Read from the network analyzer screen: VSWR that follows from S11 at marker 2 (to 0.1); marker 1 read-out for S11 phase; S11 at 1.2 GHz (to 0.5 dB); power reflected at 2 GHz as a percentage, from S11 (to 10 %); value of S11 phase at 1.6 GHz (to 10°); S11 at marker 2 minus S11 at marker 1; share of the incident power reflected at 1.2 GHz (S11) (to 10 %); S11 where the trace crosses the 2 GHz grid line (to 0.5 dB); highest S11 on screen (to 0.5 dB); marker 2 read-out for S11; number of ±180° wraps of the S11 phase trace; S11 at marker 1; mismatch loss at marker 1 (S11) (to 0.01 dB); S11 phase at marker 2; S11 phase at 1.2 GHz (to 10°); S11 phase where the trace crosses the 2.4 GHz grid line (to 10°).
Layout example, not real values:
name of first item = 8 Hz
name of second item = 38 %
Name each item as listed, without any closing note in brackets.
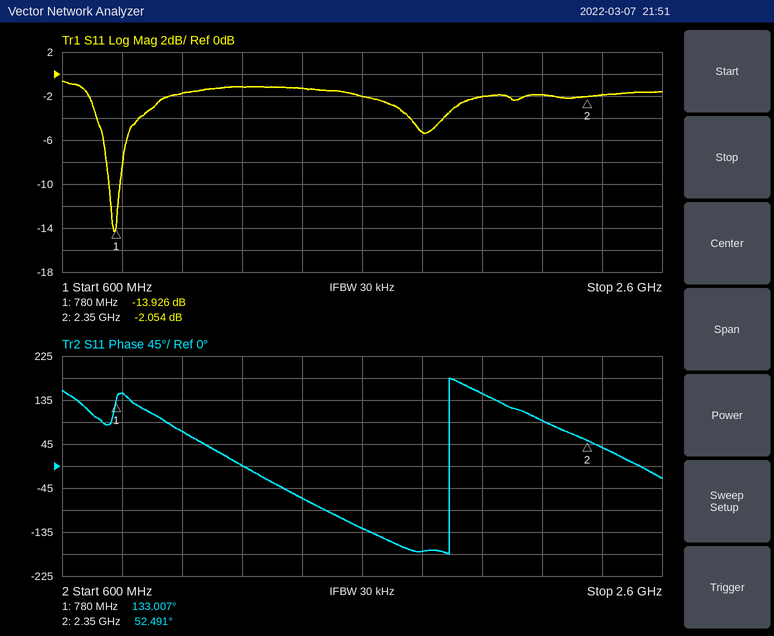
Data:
VSWR that follows from S11 at marker 2 = 8.5
marker 1 read-out for S11 phase = 133.007°
S11 at 1.2 GHz = -1.0 dB
power reflected at 2 GHz as a percentage, from S11 = 60 %
value of S11 phase at 1.6 GHz = -130°
S11 at marker 2 minus S11 at marker 1 = 11.872 dB
share of the incident power reflected at 1.2 GHz (S11) = 80 %
S11 where the trace crosses the 2 GHz grid line = -2.0 dB
highest S11 on screen = -0.5 dB
marker 2 read-out for S11 = -2.054 dB
number of ±180° wraps of the S11 phase trace = 1
S11 at marker 1 = -13.926 dB
mismatch loss at marker 1 (S11) = 0.18 dB
S11 phase at marker 2 = 52.491°
S11 phase at 1.2 GHz = 0°
S11 phase where the trace crosses the 2.4 GHz grid line = 40°
